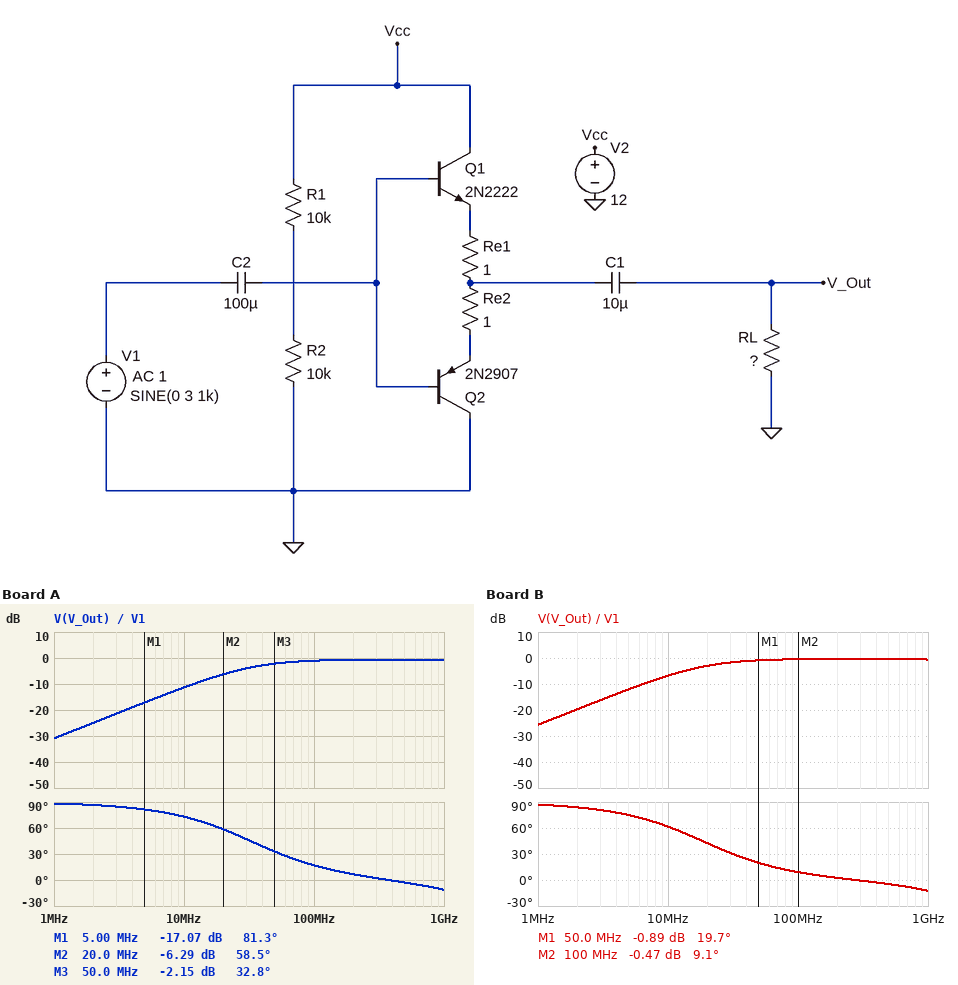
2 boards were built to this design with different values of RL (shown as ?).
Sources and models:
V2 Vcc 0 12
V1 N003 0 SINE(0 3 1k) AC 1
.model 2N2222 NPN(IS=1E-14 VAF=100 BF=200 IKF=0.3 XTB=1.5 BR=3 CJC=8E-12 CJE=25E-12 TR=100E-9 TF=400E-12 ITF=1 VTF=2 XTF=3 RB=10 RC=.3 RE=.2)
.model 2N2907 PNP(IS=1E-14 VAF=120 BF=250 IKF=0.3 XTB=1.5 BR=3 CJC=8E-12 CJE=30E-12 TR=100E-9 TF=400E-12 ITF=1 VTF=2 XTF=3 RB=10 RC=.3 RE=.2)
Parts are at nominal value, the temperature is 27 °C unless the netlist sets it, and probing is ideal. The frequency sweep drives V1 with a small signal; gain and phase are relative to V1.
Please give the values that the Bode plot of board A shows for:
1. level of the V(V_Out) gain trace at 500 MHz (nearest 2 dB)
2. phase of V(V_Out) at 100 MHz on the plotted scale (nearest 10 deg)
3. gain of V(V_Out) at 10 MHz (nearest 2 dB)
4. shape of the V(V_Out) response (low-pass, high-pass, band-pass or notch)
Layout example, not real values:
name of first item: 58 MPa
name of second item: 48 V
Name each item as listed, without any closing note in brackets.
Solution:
level of the V(V_Out) gain trace at 500 MHz: 0 dB
phase of V(V_Out) at 100 MHz on the plotted scale: 20 deg
gain of V(V_Out) at 10 MHz: -12 dB
shape of the V(V_Out) response: high-pass
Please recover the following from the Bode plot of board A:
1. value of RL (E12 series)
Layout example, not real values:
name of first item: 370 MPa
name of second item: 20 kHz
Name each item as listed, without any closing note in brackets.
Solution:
value of RL: 82 Ω
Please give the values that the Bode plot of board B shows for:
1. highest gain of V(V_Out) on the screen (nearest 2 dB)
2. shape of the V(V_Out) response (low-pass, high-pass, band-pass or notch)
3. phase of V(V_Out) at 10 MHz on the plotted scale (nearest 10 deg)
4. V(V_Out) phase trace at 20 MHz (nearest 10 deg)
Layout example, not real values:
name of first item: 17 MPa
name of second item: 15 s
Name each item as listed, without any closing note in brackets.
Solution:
highest gain of V(V_Out) on the screen: 0 dB
shape of the V(V_Out) response: high-pass
phase of V(V_Out) at 10 MHz on the plotted scale: 60 deg
V(V_Out) phase trace at 20 MHz: 40 deg
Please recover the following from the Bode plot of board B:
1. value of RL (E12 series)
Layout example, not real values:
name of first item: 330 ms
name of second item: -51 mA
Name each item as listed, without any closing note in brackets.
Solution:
value of RL: 150 Ω
